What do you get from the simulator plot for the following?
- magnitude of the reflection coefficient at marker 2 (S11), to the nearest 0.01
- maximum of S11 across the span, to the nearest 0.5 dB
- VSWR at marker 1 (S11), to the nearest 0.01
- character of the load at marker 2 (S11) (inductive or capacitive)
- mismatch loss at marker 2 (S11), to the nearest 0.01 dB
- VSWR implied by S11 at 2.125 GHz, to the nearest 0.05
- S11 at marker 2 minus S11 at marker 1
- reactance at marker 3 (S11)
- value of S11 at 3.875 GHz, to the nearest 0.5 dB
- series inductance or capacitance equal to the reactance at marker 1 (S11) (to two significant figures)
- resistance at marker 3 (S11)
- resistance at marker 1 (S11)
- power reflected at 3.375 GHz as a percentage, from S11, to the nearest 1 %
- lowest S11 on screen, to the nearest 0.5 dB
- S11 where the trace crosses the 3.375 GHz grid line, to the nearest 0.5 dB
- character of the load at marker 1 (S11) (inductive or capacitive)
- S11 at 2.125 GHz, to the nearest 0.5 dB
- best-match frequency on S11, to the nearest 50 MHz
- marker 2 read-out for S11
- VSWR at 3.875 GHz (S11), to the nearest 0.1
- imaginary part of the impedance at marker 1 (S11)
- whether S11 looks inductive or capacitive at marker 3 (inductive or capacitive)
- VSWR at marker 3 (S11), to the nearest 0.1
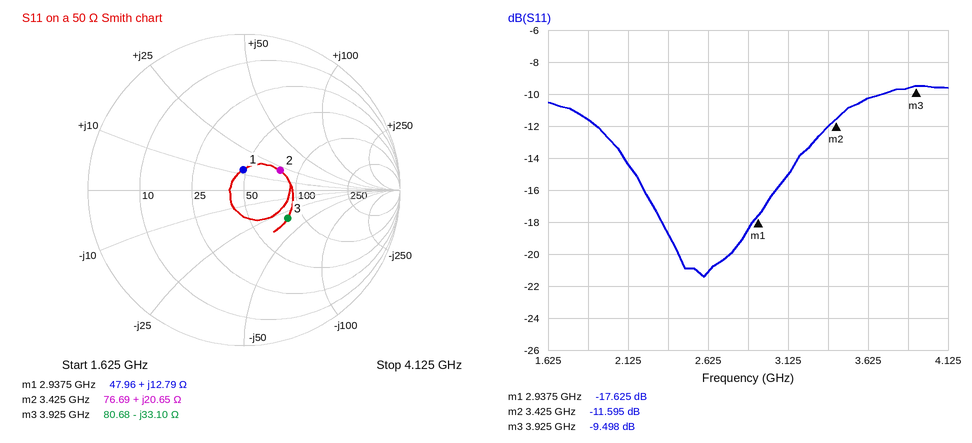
0.26
-9.5 dB
1.30
inductive
0.31 dB
1.45
6.030 dB
-33.10 Ω
-9.5 dB
690 pH
80.68 Ω
47.96 Ω
6 %
-21.5 dB
-12.0 dB
inductive
-14.5 dB
2.60 GHz
-11.595 dB
2.0
+12.79 Ω
capacitive
2.0
